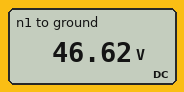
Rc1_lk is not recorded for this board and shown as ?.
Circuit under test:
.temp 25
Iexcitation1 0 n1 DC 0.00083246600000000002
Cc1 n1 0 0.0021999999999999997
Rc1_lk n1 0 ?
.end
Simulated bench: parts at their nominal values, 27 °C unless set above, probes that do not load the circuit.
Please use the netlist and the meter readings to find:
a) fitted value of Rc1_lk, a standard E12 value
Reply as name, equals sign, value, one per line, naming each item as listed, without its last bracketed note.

fitted value of Rc1_lk, a standard E12 value = 56 kΩ
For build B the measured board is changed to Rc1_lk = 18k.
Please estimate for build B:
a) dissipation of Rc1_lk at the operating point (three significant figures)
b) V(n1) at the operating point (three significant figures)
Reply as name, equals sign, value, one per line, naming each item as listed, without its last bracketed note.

dissipation of Rc1_lk at the operating point = 12.5 mW
V(n1) at the operating point = 15.0 V
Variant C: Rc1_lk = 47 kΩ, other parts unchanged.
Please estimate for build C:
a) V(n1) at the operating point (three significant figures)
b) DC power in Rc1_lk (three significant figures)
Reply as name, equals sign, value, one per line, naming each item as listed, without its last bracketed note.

V(n1) at the operating point = 39.1 V
DC power in Rc1_lk = 32.6 mW
